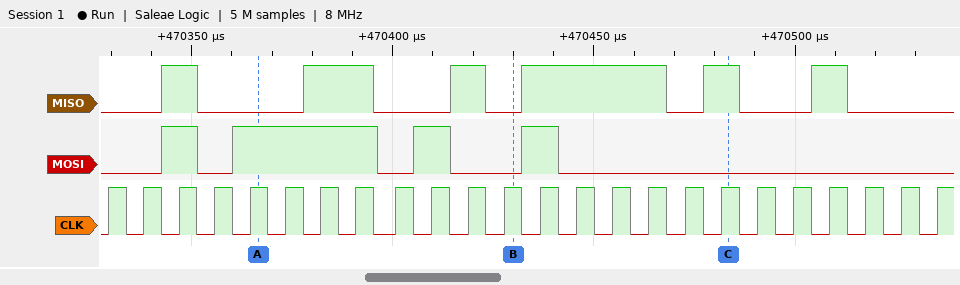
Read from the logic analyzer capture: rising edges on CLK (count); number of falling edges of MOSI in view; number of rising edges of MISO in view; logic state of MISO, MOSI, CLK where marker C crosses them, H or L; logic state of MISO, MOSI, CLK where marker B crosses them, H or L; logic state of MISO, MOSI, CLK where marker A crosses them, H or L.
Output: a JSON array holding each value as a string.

["24", "4", "6", "MISO=H, MOSI=L, CLK=H", "MISO=L, MOSI=L, CLK=H", "MISO=L, MOSI=H, CLK=H"]
